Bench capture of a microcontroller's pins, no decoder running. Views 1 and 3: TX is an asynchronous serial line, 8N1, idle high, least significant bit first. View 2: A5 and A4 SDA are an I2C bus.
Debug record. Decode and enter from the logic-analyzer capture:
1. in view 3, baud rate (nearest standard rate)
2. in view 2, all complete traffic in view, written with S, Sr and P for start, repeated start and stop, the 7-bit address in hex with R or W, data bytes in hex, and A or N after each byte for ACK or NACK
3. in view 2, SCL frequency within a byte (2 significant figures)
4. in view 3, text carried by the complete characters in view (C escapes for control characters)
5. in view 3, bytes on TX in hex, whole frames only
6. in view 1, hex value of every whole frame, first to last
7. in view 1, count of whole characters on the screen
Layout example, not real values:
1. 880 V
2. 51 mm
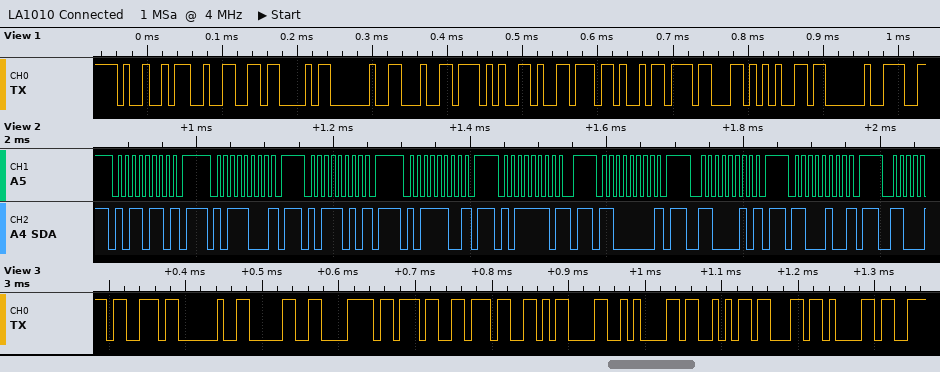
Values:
1. 115200 baud
2. S 5BW N P S 5CW N P S 5DW N P S 5EW N P S 5FW N P S 60W N P S 61W N P S 62W N P
3. 100 kHz
4. "s 0x77\r\nSca"
5. 0x73 0x20 0x30 0x78 0x37 0x37 0x0D 0x0A 0x53 0x63 0x61
6. 49 32 43 20 64 65 76 69 63 65 20
7. 11
